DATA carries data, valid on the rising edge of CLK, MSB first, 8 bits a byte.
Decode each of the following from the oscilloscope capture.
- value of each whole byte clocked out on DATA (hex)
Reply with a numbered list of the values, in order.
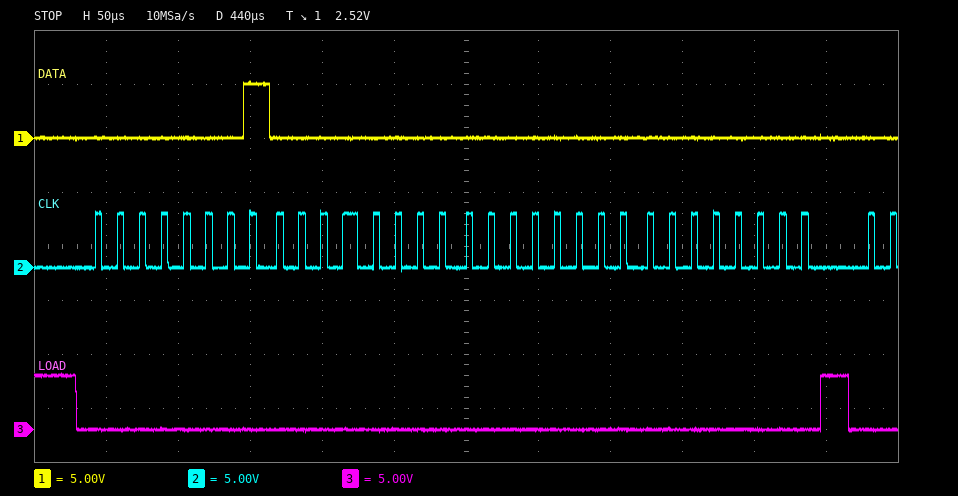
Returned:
1. 0x01 0x00 0x00 0x00
